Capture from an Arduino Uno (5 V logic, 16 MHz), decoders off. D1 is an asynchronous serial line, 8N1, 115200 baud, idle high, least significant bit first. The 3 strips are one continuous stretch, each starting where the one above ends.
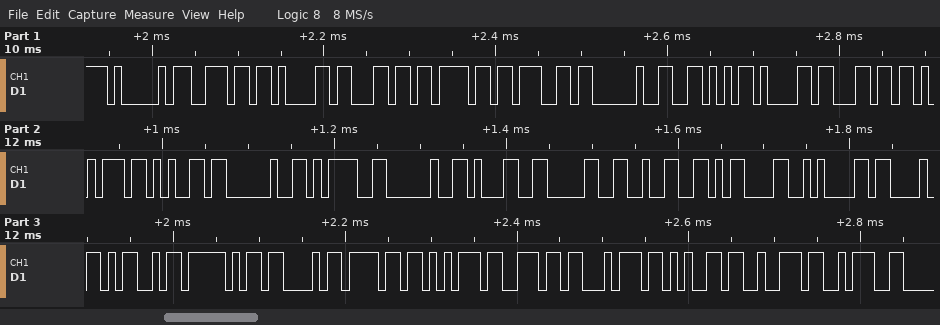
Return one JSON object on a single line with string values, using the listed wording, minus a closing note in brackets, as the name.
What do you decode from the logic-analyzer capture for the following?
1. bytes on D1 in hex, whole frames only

{"bytes on D1 in hex, whole frames only": "41 6E 61 6C 6F 67 20 56 61 6C 75 65 20 3D 20 31 30 32 0D 0A 43 4D 5F 43 6F 75 6E 74 65 72 3A"}
